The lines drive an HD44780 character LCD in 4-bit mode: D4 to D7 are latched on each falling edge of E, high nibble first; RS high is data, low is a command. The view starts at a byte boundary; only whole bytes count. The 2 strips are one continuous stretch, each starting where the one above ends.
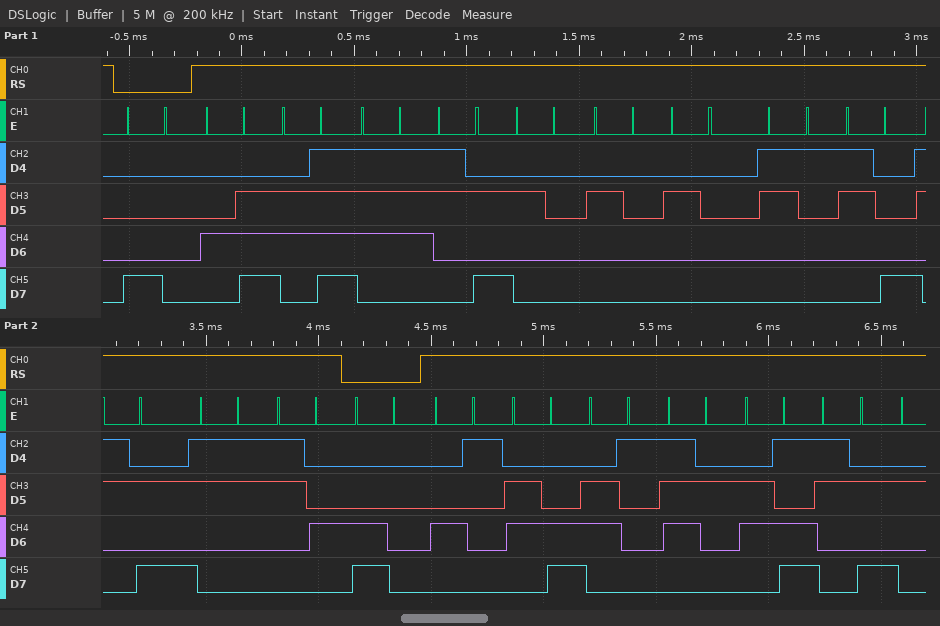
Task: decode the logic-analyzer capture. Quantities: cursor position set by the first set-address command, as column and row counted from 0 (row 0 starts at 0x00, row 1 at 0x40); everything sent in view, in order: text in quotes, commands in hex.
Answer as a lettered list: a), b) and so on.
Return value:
a) column 0, row 0
b) 0x80 "Now:   18:34" 0xC0 "Alarm:"
